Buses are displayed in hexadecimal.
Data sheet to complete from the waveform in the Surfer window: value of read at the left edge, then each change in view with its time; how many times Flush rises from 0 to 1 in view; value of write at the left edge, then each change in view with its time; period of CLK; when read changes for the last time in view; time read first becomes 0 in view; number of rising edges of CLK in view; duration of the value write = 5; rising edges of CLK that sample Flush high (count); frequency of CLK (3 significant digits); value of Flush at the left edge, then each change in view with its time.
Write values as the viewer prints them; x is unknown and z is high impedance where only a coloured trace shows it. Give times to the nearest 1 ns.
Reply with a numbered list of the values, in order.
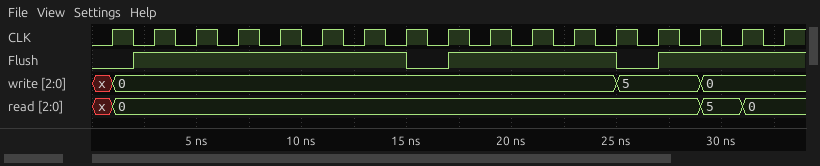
1. x, 0 at 1 ns, 5 at 29 ns, 0 at 31 ns
2. 3
3. x, 0 at 1 ns, 5 at 25 ns, 0 at 29 ns
4. 2 ns
5. 31 ns
6. 1 ns
7. 17
8. 4 ns
9. 14
10. 500 MHz
11. 0, 1 at 2 ns, 0 at 15 ns, 1 at 17 ns, 0 at 25 ns, 1 at 27 ns
